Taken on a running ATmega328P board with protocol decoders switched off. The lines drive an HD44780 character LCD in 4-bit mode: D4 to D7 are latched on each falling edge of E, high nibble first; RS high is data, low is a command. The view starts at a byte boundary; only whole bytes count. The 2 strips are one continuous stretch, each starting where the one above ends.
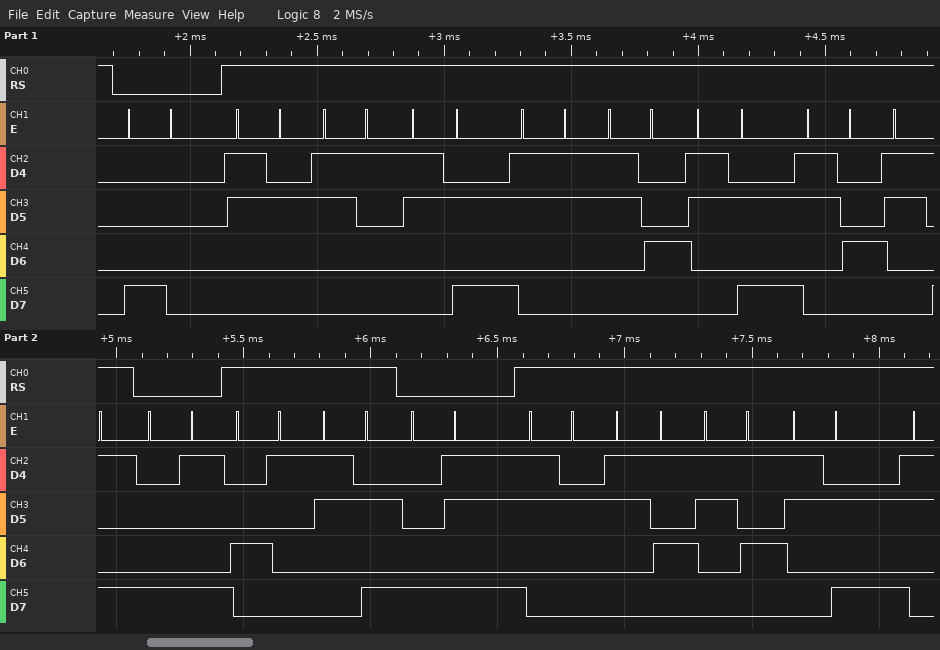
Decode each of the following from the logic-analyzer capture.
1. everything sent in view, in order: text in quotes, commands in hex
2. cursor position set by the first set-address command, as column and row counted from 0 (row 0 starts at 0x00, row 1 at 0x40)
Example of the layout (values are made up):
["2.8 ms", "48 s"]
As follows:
["0x80 \"21:34:49\" 0x89 \"A:\" 0x8B \"255:\"", "column 0, row 0"]
